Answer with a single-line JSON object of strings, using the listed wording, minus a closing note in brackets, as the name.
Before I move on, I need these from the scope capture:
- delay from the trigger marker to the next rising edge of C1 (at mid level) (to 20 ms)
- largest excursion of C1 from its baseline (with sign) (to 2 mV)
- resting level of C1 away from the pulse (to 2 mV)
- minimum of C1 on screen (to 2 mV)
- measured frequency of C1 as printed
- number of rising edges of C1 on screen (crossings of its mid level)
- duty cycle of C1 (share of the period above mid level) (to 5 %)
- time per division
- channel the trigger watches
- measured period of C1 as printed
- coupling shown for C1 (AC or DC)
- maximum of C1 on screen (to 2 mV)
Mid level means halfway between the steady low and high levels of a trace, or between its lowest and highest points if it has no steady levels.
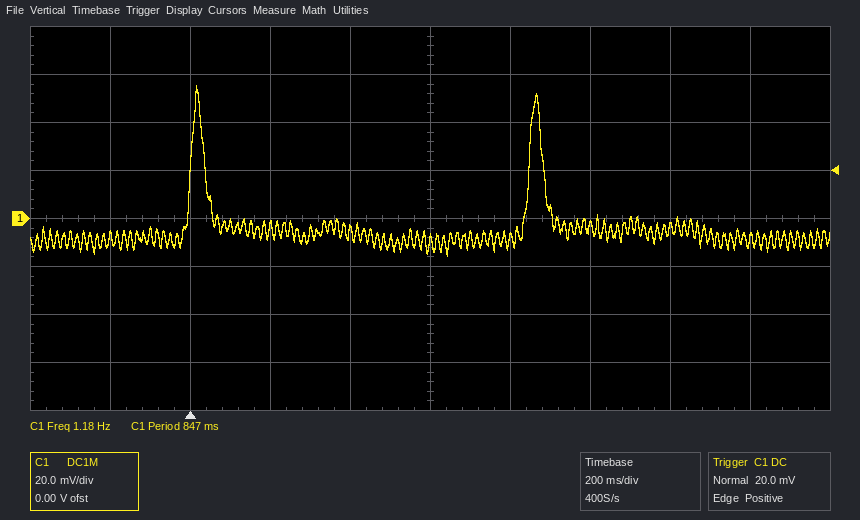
{"delay from the trigger marker to the next rising edge of C1 (at mid level)": "840 ms", "largest excursion of C1 from its baseline (with sign)": "+62 mV", "resting level of C1 away from the pulse": "-6 mV", "minimum of C1 on screen": "-16 mV", "measured frequency of C1 as printed": "1.18 Hz", "number of rising edges of C1 on screen": "2", "duty cycle of C1 (share of the period above mid level)": "5 %", "time per division": "200 ms", "channel the trigger watches": "C1", "measured period of C1 as printed": "847 ms", "coupling shown for C1": "DC", "maximum of C1 on screen": "56 mV"}
